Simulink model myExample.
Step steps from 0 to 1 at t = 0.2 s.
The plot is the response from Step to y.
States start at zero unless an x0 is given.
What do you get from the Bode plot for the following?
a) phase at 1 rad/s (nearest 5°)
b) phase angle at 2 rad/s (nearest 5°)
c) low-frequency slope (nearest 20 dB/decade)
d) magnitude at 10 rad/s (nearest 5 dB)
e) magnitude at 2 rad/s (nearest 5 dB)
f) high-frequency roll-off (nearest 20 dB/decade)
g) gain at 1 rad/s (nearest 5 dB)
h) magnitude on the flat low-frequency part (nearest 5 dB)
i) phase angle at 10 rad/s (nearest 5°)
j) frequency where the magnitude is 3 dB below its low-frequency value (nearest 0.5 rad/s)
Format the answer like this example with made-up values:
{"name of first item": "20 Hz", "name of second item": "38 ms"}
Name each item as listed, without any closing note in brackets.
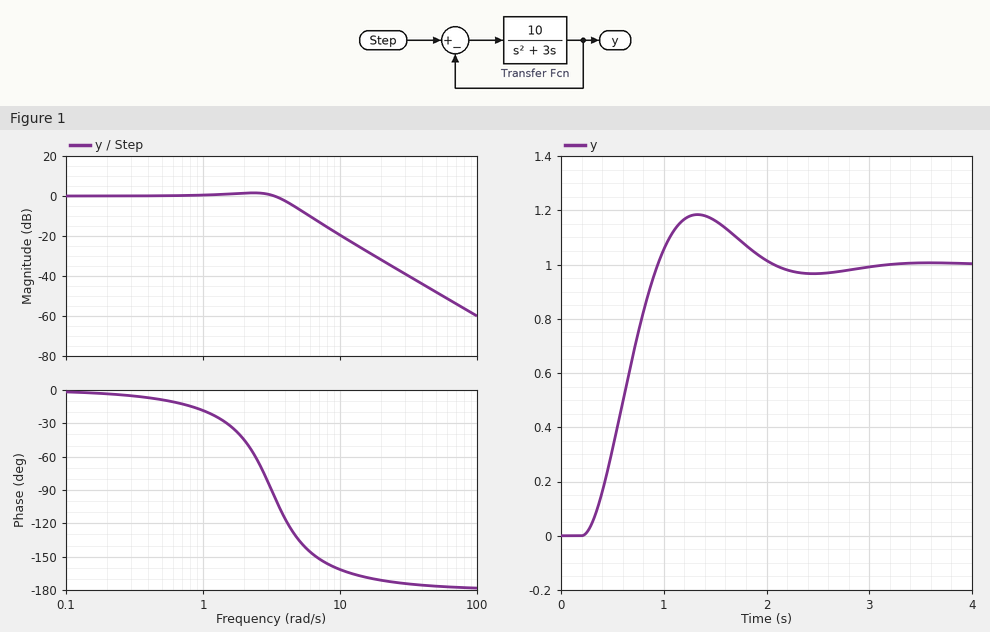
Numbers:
{"phase at 1 rad/s": "-20°", "phase angle at 2 rad/s": "-45°", "low-frequency slope": "0 dB/decade", "magnitude at 10 rad/s": "-20 dB", "magnitude at 2 rad/s": "0 dB", "high-frequency roll-off": "-40 dB/decade", "gain at 1 rad/s": "0 dB", "magnitude on the flat low-frequency part": "0 dB", "phase angle at 10 rad/s": "-160°", "frequency where the magnitude is 3 dB below its low-frequency value": "4.0 rad/s"}
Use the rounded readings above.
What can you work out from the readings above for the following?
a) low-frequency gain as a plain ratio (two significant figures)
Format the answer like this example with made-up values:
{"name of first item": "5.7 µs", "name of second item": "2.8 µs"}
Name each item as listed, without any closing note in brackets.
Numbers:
{"low-frequency gain as a plain ratio": "1.0"}
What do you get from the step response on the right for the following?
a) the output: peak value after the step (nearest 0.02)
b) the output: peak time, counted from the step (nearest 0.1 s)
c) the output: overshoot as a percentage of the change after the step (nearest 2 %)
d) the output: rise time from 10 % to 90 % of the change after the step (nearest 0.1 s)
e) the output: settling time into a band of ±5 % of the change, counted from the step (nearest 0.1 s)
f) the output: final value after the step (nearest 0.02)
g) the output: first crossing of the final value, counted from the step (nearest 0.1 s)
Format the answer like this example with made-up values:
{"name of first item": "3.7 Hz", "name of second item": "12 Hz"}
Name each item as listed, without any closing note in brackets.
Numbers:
{"the output: peak value after the step": "1.18", "the output: peak time, counted from the step": "1.1 s", "the output: overshoot as a percentage of the change after the step": "18 %", "the output: rise time from 10 % to 90 % of the change after the step": "0.5 s", "the output: settling time into a band of ±5 % of the change, counted from the step": "1.7 s", "the output: final value after the step": "1.00", "the output: first crossing of the final value, counted from the step": "0.7 s"}
